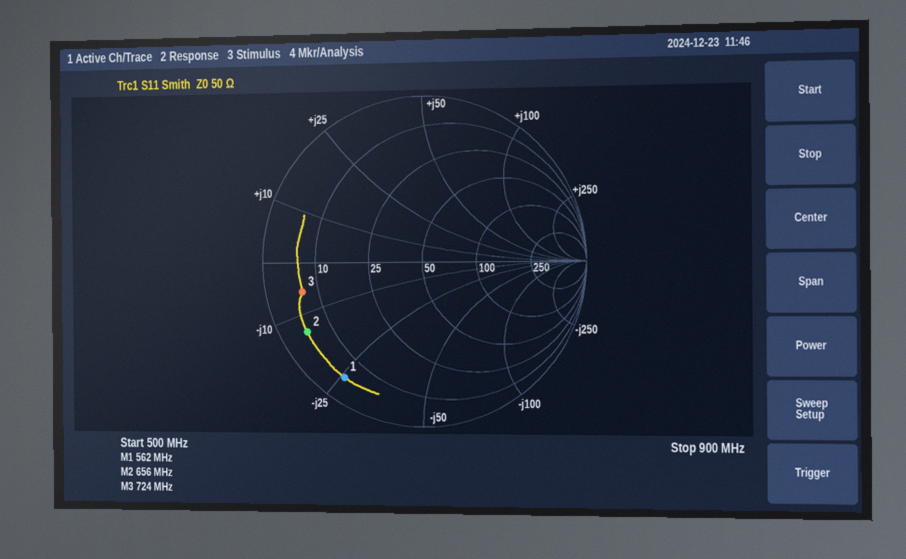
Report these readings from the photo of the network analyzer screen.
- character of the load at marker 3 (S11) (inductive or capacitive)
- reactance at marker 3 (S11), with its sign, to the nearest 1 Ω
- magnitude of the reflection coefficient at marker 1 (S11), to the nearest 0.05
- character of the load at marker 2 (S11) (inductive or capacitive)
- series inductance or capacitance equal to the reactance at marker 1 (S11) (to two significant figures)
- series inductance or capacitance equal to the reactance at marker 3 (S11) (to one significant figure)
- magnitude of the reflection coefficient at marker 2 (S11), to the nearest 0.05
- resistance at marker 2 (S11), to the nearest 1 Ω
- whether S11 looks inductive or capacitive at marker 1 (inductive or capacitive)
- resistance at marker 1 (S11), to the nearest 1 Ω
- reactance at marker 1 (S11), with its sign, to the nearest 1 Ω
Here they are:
capacitive
-6 Ω
0.85
capacitive
11 pF
40 pF
0.85
5 Ω
capacitive
5 Ω
-26 Ω
